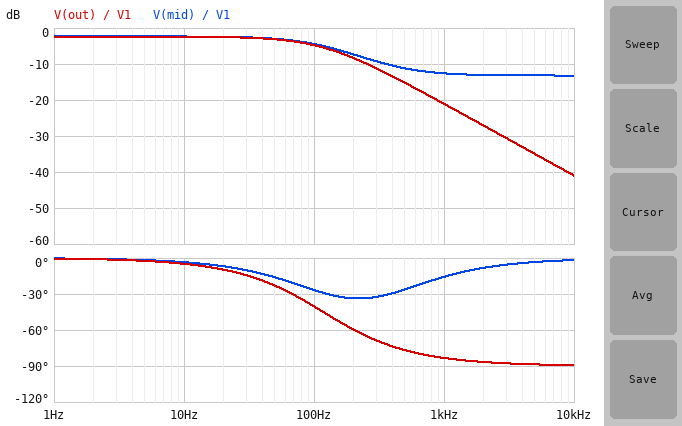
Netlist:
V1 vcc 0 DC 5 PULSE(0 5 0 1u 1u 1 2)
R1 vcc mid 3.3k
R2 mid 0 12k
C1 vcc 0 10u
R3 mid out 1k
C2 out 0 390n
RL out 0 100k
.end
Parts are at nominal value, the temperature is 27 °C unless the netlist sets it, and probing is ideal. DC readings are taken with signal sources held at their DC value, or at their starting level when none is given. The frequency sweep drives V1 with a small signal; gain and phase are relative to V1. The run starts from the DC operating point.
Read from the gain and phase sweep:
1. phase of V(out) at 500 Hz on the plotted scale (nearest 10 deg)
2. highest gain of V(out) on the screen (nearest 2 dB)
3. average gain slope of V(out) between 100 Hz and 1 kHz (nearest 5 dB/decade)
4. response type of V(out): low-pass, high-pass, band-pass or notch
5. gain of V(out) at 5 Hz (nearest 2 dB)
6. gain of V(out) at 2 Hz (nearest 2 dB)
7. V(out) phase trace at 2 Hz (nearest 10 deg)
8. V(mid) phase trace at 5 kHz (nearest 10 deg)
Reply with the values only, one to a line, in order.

-80 deg
-2 dB
-15 dB/decade
low-pass
-2 dB
-2 dB
0 deg
0 deg
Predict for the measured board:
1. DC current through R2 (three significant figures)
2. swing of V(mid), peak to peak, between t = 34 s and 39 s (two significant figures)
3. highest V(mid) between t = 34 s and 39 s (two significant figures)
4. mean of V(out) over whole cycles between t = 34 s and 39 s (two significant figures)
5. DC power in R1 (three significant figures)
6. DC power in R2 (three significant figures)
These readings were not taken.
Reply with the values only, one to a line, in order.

319 µA
3.8 V
3.8 V
1.9 V
419 µW
1.22 mW
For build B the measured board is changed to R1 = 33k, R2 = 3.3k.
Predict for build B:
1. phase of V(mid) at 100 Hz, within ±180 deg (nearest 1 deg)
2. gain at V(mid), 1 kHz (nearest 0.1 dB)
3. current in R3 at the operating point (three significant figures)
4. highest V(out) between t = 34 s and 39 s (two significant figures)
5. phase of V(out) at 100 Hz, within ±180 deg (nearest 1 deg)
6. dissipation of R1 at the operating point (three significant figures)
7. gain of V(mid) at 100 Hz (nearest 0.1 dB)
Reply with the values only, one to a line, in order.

-30 deg
-32.2 dB
4.37 µA
440 mV
-43 deg
630 µW
-23.6 dB
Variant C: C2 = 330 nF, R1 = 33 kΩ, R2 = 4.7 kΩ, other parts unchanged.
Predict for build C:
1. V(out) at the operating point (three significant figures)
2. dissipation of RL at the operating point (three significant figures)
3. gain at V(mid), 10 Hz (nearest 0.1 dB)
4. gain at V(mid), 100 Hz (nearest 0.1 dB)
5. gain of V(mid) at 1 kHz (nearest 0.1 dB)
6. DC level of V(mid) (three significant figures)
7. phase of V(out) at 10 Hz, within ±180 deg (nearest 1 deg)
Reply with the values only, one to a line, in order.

593 mV
3.52 µW
-18.5 dB
-21.3 dB
-31.4 dB
599 mV
-6 deg
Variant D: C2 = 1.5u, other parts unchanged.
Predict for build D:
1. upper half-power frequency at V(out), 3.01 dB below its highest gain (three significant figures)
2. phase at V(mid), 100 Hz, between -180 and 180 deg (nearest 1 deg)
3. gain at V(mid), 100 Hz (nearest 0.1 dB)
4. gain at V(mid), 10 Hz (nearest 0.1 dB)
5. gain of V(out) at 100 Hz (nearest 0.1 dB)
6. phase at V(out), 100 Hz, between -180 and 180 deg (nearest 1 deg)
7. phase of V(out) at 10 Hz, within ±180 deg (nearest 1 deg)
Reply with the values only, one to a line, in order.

30.6 Hz
-30 deg
-10.3 dB
-2.7 dB
-13.1 dB
-73 deg
-18 deg
